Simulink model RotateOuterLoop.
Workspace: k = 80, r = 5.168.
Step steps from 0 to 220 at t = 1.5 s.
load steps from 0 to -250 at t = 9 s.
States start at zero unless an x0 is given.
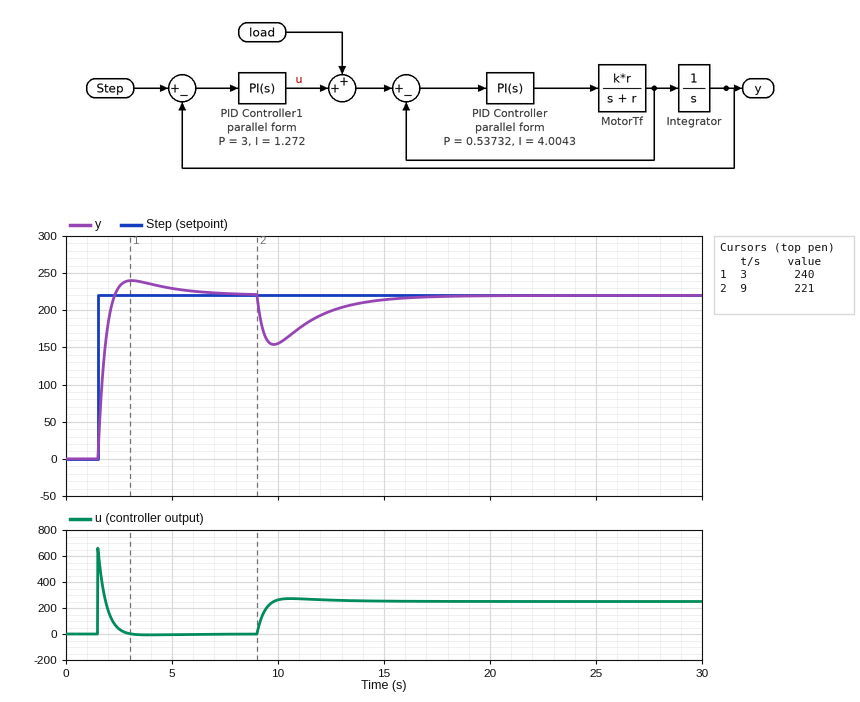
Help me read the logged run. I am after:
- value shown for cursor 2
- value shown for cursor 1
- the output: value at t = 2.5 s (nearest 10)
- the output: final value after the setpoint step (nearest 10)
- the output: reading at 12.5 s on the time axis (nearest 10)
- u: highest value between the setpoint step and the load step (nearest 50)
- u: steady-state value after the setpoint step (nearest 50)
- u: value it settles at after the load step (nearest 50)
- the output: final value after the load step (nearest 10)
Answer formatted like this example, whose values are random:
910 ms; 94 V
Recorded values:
221; 240; 230; 220; 200; 650; 0; 250; 220
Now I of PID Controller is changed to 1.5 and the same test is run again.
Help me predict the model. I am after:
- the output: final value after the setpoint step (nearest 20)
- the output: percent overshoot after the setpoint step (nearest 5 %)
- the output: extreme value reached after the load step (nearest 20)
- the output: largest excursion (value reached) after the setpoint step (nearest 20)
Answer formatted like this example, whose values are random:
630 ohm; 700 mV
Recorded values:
220; 10 %; 160; 240
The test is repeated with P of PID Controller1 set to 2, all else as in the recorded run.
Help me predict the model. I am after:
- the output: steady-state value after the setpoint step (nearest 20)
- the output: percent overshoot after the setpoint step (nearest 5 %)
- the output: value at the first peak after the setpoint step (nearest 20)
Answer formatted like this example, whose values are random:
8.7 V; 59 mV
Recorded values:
220; 15 %; 260
